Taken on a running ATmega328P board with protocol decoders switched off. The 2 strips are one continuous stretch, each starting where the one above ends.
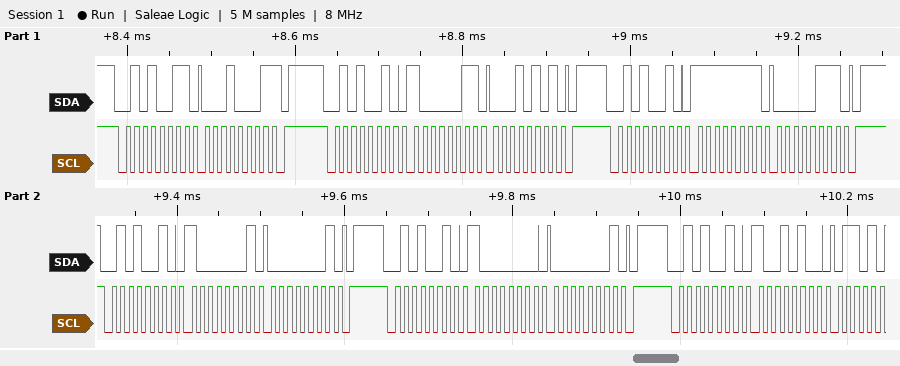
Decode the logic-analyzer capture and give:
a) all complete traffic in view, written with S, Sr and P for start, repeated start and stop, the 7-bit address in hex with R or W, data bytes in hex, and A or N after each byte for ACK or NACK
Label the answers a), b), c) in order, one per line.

a) S 29R A 11 N P S 29W A 83 A 15 A P S 29W A FF A 07 A P S 29W A 81 A 01 A P S 29W A 80 A 01 A P S 29W A 94 A
